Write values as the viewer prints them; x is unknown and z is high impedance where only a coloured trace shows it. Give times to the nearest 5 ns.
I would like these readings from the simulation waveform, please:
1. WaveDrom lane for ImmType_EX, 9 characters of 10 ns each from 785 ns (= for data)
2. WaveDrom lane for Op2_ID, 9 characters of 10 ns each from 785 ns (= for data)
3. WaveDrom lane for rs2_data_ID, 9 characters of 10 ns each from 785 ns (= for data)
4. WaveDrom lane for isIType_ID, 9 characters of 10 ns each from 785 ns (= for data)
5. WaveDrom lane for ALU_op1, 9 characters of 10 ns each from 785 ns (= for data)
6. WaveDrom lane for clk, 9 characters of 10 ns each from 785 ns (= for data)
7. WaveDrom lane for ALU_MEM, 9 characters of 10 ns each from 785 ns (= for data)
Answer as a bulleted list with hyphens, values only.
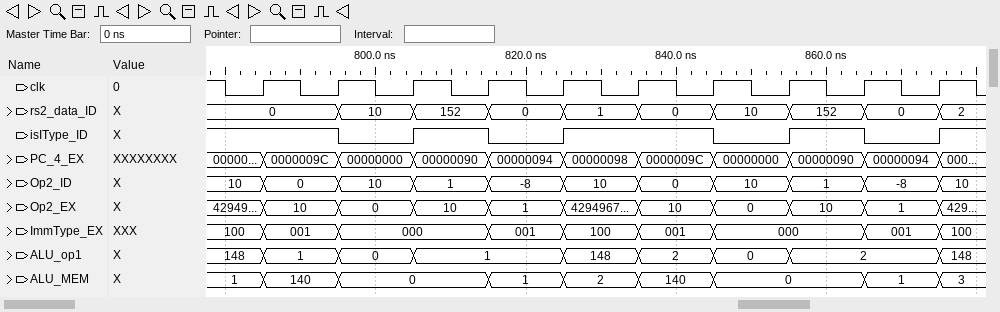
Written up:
- {name: 'ImmType_EX', wave: '==.====.=', data: '001 000 001 100 001 000 001'}
- {name: 'Op2_ID', wave: '=========', data: '0 10 1 -8 10 0 10 1 -8'}
- {name: 'rs2_data_ID', wave: '=========', data: '0 10 152 0 1 0 10 152 0'}
- {name: 'isIType_ID', wave: '10101.010'}
- {name: 'ALU_op1', wave: '===.====.', data: '1 0 1 148 2 0 2'}
- {name: 'clk', wave: 'p........'}
- {name: 'ALU_MEM', wave: '==.====.=', data: '140 0 1 2 140 0 1'}
